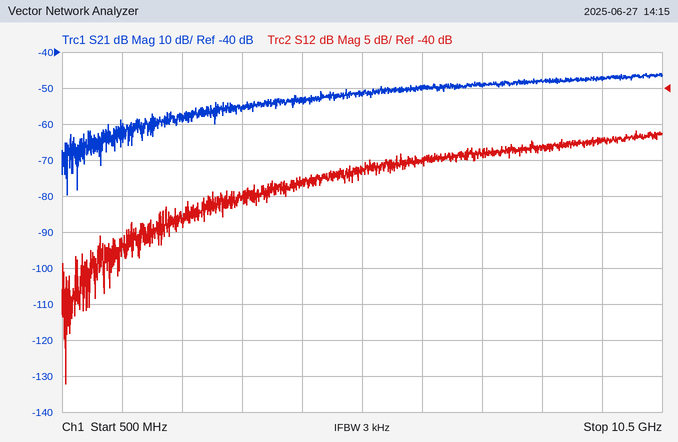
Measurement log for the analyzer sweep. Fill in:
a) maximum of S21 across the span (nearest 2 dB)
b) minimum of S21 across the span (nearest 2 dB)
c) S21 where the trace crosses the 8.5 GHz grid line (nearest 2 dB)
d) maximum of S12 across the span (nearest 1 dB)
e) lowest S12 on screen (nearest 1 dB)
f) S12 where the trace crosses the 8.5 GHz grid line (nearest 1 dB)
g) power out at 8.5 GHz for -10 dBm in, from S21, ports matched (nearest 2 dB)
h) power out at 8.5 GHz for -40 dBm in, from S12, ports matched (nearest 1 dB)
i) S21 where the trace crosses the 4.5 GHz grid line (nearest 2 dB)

-46 dB
-80 dB
-48 dB
-46 dB
-81 dB
-48 dB
-58 dBm
-88 dBm
-54 dB
